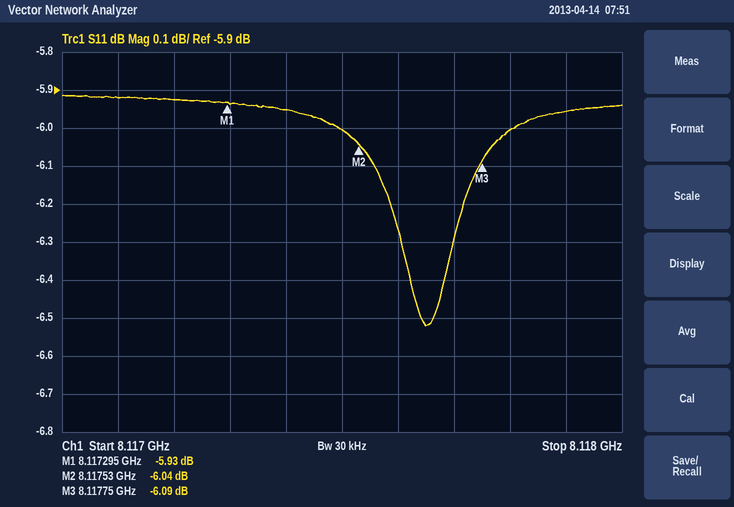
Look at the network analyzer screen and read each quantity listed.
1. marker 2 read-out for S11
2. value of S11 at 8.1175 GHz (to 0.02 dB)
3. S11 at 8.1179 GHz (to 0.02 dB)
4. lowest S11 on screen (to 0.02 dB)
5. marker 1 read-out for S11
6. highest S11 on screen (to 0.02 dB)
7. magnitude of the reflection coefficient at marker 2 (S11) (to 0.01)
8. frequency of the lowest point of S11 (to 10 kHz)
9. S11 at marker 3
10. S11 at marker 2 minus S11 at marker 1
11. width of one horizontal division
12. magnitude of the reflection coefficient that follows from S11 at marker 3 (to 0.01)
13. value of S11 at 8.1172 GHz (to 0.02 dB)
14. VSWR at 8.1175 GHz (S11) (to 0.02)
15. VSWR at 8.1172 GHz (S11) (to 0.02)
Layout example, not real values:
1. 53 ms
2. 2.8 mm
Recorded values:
1. -6.04 dB
2. -6.00 dB
3. -5.96 dB
4. -6.52 dB
5. -5.93 dB
6. -5.92 dB
7. 0.50
8. 8.11765 GHz
9. -6.09 dB
10. -0.11 dB
11. 100 kHz
12. 0.50
13. -5.92 dB
14. 3.00
15. 3.04
